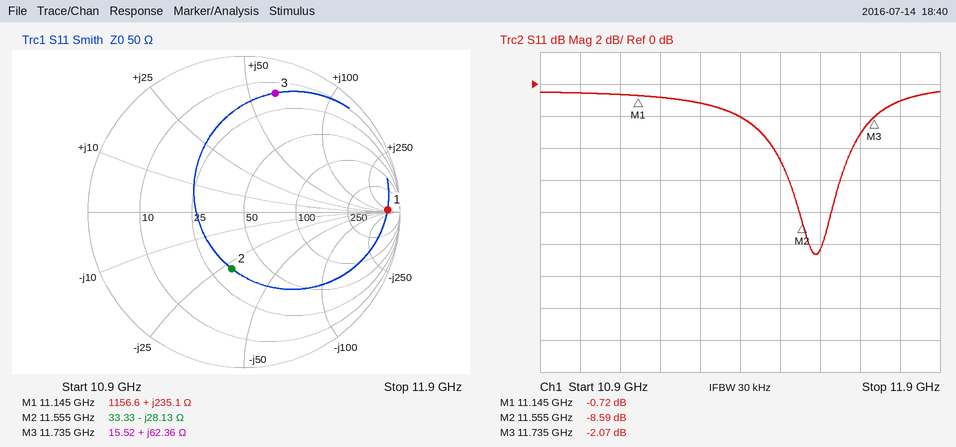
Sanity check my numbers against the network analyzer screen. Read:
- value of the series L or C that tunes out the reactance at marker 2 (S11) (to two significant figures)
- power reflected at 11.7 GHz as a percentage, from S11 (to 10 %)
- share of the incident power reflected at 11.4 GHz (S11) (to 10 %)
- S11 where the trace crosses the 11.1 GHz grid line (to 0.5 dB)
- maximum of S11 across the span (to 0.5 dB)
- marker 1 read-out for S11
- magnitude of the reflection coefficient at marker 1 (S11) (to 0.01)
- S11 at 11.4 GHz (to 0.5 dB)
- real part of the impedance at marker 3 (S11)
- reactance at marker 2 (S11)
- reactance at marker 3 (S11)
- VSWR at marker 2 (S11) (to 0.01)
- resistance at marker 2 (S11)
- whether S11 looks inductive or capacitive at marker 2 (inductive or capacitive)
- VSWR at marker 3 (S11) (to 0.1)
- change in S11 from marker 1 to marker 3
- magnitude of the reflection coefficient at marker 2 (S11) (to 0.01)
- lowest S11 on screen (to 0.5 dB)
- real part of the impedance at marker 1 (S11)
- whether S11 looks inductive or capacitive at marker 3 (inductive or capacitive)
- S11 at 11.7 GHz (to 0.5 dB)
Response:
390 pH
50 %
60 %
-0.5 dB
-0.5 dB
-0.72 dB
0.92
-2.0 dB
15.52 Ω
-28.13 Ω
+62.36 Ω
2.18
33.33 Ω
capacitive
8.4
-1.35 dB
0.37
-10.5 dB
1156.6 Ω
inductive
-3.0 dB
